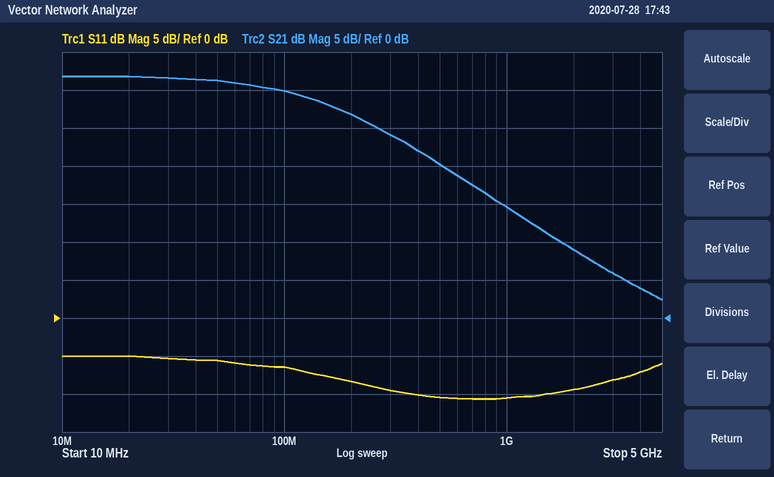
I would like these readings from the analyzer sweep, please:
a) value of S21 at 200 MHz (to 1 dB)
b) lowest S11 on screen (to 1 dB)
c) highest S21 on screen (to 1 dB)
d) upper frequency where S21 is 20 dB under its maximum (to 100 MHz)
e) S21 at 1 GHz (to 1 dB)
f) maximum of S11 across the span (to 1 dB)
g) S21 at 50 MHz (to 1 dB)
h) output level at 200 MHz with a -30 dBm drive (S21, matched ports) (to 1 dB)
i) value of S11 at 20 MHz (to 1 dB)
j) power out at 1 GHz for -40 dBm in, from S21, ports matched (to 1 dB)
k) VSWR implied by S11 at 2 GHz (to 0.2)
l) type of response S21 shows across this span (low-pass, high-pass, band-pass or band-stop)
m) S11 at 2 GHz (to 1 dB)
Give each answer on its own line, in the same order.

27 dB
-11 dB
32 dB
1.4 GHz
15 dB
-5 dB
31 dB
-3 dBm
-5 dB
-25 dBm
2.0
low-pass
-9 dB
